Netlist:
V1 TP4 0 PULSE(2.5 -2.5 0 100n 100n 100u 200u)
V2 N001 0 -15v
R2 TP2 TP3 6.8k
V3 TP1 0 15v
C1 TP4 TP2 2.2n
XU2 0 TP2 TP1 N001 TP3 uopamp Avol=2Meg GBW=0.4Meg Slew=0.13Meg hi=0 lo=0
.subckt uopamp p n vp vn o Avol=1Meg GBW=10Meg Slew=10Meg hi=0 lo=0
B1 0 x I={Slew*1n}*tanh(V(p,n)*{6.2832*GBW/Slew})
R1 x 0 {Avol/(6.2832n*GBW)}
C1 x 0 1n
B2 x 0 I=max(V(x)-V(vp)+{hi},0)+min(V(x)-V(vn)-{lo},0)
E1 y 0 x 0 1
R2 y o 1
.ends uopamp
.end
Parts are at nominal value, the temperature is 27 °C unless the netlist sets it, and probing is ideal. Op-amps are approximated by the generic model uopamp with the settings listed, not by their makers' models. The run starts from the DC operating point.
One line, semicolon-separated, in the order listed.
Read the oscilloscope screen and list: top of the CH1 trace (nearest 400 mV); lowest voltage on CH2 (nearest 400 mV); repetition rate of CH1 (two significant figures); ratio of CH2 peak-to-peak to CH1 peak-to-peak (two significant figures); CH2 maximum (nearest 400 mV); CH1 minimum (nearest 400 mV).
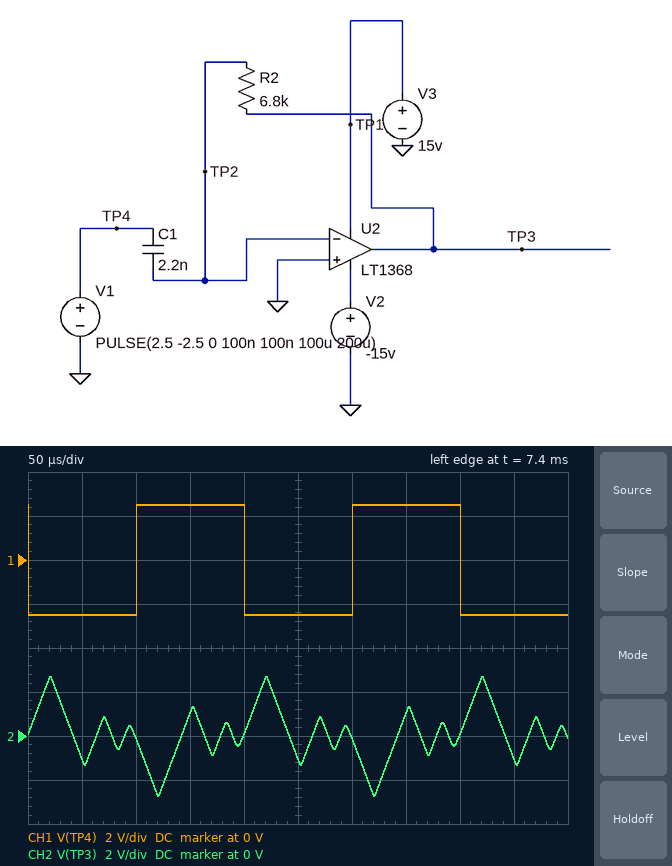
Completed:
2.4 V; -2.8 V; 5.0 kHz; 1.1; 2.8 V; -2.4 V
